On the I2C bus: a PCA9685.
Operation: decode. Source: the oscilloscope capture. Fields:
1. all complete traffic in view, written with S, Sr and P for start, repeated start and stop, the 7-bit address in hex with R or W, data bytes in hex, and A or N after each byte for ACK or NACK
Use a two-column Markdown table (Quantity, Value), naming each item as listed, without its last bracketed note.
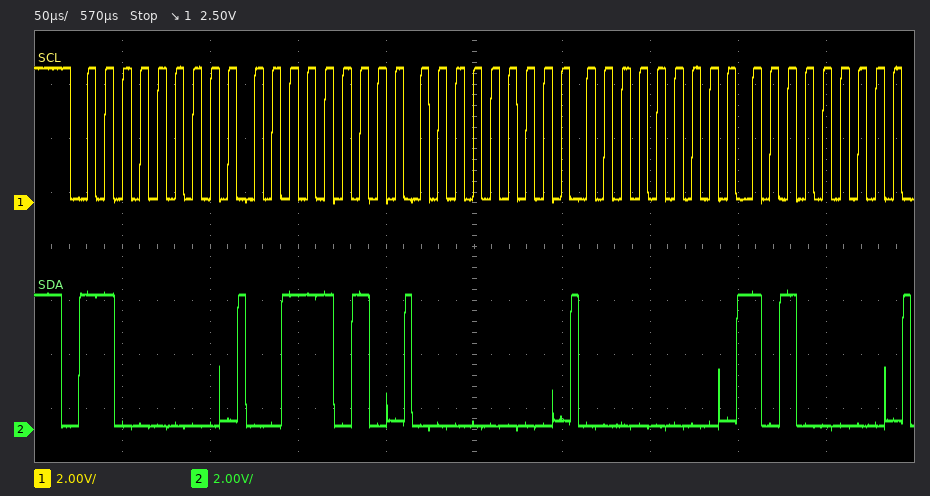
| Quantity | Value |
|---|---|
| all complete traffic in view, written with S, Sr and P for start, repeated start and stop, the 7-bit address in hex with R or W, data bytes in hex, and A or N after each byte for ACK or NACK | S 60W A 3A A 00 A 00 A A0 A |
